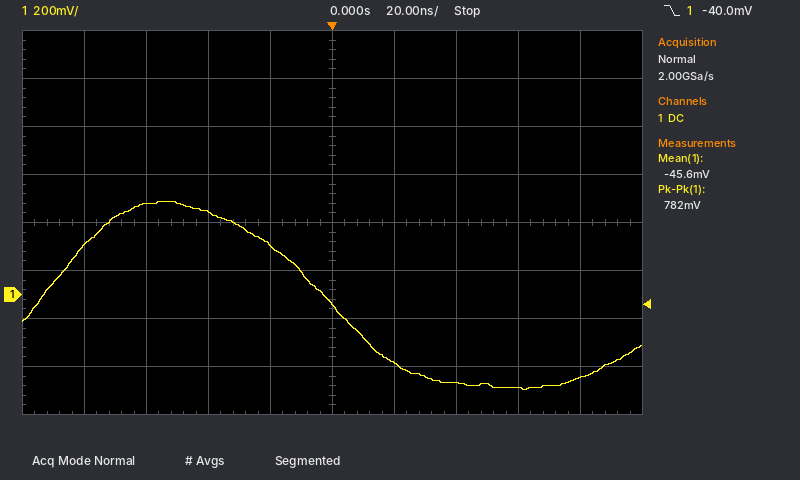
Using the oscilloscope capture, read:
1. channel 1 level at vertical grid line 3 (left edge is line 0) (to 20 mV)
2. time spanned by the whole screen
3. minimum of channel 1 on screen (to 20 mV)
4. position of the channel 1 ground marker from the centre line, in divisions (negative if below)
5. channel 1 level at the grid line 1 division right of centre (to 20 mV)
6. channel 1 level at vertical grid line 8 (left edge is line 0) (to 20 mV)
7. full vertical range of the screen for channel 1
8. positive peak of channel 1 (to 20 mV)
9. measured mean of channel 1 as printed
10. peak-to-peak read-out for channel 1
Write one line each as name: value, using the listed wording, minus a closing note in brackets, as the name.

channel 1 level at vertical grid line 3 (left edge is line 0): 340 mV
time spanned by the whole screen: 200 ns
minimum of channel 1 on screen: -400 mV
position of the channel 1 ground marker from the centre line, in divisions: -1.5 div
channel 1 level at the grid line 1 division right of centre: -280 mV
channel 1 level at vertical grid line 8 (left edge is line 0): -380 mV
full vertical range of the screen for channel 1: 1.6 V
positive peak of channel 1: 380 mV
measured mean of channel 1 as printed: -45.6 mV
peak-to-peak read-out for channel 1: 782 mV
